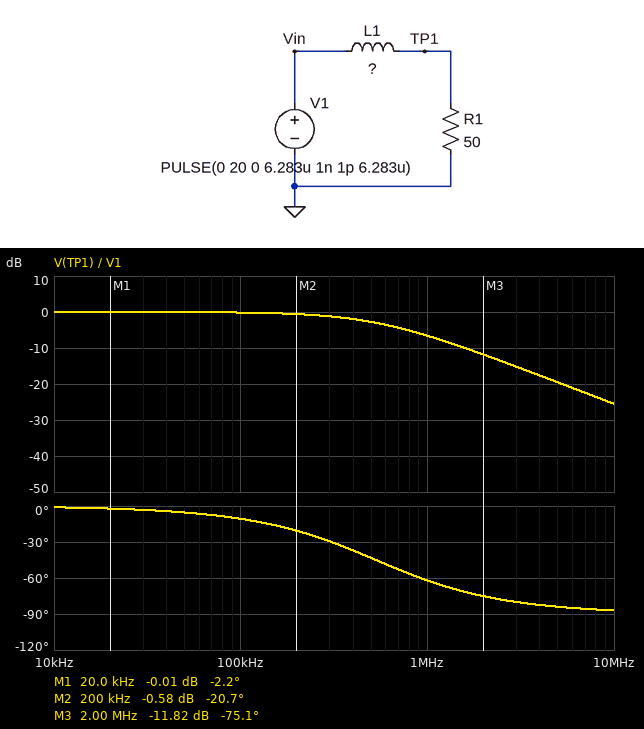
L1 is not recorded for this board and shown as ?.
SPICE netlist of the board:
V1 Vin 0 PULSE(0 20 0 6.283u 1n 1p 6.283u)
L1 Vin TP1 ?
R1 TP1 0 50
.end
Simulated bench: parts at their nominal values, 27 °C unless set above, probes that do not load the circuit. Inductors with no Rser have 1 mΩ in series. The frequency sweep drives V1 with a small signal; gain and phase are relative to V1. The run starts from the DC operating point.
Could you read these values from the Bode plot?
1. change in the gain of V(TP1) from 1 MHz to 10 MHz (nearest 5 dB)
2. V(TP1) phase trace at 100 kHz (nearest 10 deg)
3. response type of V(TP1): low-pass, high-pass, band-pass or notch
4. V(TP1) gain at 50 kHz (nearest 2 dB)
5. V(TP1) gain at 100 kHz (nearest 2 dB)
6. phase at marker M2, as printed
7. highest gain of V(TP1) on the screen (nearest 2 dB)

-20 dB
-10 deg
low-pass
0 dB
0 dB
-20.7 deg
0 dB
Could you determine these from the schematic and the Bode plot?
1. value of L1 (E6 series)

15 µH
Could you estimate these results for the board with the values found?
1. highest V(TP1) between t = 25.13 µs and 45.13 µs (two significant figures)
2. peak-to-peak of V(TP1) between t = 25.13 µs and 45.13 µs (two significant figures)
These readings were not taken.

19 V
16 V
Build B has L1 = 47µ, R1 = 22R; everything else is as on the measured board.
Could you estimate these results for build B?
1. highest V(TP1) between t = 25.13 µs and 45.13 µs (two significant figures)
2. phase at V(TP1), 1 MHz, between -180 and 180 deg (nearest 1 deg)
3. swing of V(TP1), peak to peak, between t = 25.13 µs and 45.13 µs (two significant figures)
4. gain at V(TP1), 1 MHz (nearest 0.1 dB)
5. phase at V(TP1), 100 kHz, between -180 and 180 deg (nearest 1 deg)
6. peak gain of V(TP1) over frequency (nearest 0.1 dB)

14 V
-86 deg
6.6 V
-22.6 dB
-53 deg
0 dB
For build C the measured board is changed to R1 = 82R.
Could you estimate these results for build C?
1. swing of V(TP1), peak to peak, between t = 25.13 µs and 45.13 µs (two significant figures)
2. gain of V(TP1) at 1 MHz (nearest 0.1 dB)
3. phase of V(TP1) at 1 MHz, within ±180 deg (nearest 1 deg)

17 V
-3.7 dB
-49 deg
